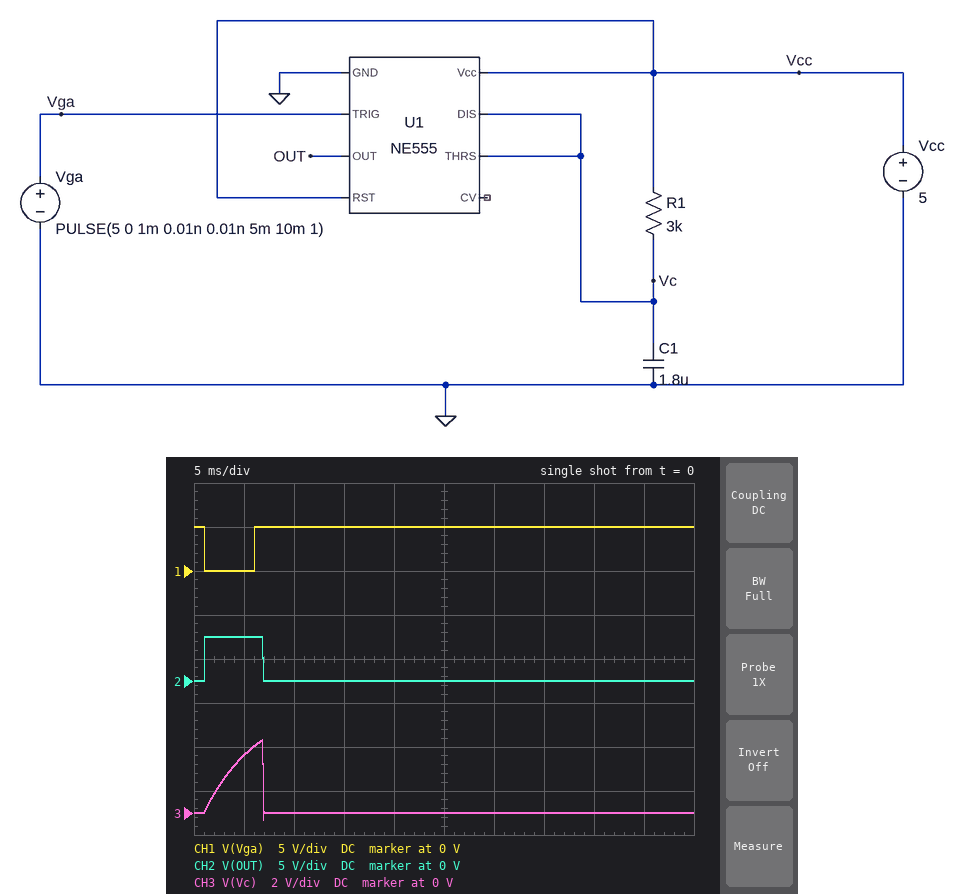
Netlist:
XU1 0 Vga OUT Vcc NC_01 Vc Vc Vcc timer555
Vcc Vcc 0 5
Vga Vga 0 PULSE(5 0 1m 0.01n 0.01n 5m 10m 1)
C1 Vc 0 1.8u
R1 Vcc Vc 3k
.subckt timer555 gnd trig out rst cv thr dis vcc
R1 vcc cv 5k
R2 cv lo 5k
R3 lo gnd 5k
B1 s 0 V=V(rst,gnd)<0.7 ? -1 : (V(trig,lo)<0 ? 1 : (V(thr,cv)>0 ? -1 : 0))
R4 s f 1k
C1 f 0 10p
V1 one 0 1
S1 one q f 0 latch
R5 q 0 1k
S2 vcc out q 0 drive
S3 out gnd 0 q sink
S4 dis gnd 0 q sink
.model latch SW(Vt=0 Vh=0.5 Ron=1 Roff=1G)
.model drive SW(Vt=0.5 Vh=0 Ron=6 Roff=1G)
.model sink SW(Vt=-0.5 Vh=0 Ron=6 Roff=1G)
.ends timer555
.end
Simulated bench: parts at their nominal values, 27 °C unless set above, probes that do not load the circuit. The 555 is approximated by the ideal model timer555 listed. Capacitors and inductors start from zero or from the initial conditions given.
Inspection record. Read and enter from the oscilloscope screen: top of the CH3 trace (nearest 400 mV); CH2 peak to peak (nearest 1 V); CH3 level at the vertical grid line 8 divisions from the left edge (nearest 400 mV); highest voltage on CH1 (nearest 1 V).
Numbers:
3.2 V
5 V
0 V
5 V
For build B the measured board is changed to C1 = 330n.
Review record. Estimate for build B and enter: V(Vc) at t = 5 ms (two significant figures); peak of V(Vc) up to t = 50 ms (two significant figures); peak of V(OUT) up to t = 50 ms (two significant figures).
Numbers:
4.9 V
5.0 V
5.0 V
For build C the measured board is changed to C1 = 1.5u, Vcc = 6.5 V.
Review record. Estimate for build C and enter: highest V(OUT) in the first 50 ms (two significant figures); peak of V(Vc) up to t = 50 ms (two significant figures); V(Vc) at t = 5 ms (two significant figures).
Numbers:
6.5 V
4.4 V
3.8 V
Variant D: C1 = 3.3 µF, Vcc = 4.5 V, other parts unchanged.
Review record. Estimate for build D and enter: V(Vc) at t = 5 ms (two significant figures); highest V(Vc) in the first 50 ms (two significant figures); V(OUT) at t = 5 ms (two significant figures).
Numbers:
1.5 V
3.0 V
4.5 V
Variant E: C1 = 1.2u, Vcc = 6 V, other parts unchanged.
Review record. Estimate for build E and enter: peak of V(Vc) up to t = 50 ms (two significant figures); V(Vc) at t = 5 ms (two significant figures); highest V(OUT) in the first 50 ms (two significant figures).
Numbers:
4.5 V
4.0 V
6.0 V
